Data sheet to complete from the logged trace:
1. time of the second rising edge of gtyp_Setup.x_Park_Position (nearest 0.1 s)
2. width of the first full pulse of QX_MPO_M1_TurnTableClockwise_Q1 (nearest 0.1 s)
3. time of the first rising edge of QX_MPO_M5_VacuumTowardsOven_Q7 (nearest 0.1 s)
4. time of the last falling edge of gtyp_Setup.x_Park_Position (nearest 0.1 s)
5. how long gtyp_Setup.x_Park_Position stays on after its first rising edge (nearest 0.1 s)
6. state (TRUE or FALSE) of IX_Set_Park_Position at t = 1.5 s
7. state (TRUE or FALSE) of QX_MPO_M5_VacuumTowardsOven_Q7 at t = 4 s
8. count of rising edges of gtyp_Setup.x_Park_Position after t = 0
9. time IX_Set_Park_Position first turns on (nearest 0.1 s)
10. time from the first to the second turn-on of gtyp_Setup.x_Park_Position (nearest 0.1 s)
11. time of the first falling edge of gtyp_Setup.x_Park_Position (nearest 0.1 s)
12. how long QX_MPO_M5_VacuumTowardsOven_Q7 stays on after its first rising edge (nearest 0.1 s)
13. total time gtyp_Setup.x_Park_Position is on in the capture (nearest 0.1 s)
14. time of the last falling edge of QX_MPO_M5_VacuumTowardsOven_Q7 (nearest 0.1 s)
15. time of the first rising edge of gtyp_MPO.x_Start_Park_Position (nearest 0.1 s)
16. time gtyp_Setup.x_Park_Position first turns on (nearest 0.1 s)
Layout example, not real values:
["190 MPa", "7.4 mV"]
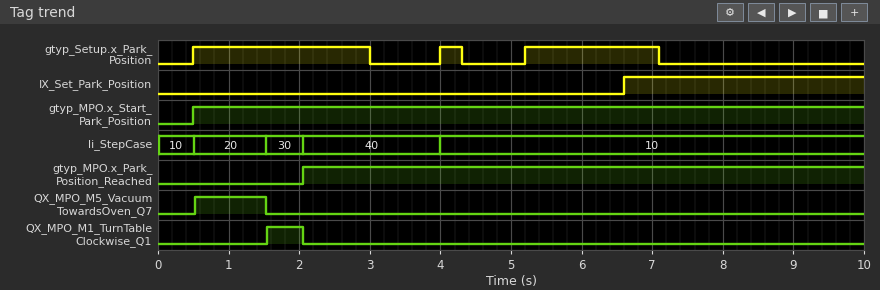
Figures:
["4.0 s", "0.5 s", "0.5 s", "7.1 s", "2.5 s", "FALSE", "FALSE", "3", "6.6 s", "3.5 s", "3.0 s", "1.0 s", "4.7 s", "1.5 s", "0.5 s", "0.5 s"]
